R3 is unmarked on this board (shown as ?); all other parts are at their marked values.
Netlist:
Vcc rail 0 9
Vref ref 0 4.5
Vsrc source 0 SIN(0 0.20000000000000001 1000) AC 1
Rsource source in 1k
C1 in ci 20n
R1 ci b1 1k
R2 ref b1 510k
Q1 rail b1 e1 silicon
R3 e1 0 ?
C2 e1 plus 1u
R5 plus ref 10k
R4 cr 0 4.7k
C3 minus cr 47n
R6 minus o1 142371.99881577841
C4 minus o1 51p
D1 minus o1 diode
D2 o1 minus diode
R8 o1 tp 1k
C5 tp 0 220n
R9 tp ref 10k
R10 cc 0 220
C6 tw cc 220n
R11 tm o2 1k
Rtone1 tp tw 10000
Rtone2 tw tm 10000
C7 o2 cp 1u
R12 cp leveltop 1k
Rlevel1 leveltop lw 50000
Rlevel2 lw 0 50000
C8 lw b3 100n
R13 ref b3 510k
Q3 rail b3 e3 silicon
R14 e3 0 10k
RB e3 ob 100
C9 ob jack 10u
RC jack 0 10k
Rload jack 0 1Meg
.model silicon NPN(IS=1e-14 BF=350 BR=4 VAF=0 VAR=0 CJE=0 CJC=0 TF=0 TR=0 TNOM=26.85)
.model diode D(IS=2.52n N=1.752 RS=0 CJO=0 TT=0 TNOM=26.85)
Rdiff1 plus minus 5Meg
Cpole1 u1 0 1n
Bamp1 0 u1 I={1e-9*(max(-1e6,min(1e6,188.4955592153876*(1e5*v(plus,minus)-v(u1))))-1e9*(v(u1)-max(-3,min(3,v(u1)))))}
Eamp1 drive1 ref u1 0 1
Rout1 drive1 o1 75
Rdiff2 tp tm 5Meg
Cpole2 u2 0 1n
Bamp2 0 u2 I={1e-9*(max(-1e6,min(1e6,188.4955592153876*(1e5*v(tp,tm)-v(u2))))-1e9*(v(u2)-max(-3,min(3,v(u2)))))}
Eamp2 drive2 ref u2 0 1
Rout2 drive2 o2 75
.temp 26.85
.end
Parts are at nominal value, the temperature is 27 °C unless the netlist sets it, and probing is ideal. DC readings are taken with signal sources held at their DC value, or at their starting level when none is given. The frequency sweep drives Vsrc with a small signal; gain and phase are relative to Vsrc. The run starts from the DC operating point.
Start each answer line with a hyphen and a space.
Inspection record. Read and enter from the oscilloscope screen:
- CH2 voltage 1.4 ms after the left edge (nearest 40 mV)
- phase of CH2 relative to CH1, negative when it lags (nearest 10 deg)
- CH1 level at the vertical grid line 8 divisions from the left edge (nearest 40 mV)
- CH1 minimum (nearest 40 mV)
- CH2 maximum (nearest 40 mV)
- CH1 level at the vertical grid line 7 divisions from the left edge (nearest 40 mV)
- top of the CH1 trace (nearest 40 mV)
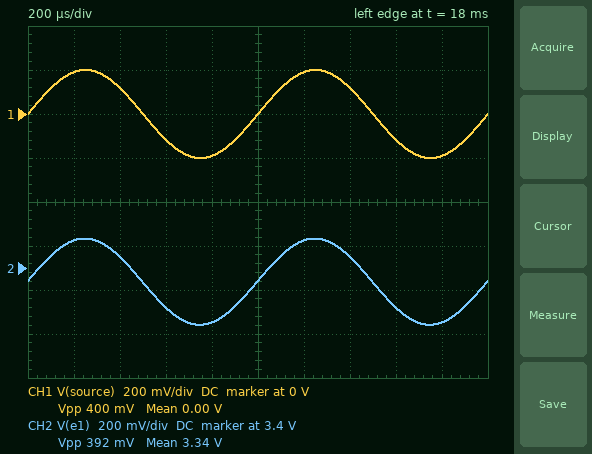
- 3.44 V
- 0 deg
- -120 mV
- -200 mV
- 3.52 V
- 120 mV
- 200 mV
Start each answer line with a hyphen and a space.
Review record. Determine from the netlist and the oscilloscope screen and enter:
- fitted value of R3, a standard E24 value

- 9.1 kΩ
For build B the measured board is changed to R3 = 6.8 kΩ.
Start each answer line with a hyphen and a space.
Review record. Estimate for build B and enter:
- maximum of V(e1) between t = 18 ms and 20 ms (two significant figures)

- 3.4 V
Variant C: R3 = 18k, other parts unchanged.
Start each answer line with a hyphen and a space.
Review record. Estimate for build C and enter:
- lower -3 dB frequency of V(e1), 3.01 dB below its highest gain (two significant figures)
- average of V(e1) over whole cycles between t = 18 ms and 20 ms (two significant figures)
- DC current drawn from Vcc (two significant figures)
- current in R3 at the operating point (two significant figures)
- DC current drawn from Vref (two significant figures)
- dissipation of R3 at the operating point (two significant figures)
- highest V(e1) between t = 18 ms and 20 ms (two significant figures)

- 19 Hz
- 3.6 V
- 540 µA
- 200 µA
- 1.5 µA
- 720 µW
- 3.8 V
